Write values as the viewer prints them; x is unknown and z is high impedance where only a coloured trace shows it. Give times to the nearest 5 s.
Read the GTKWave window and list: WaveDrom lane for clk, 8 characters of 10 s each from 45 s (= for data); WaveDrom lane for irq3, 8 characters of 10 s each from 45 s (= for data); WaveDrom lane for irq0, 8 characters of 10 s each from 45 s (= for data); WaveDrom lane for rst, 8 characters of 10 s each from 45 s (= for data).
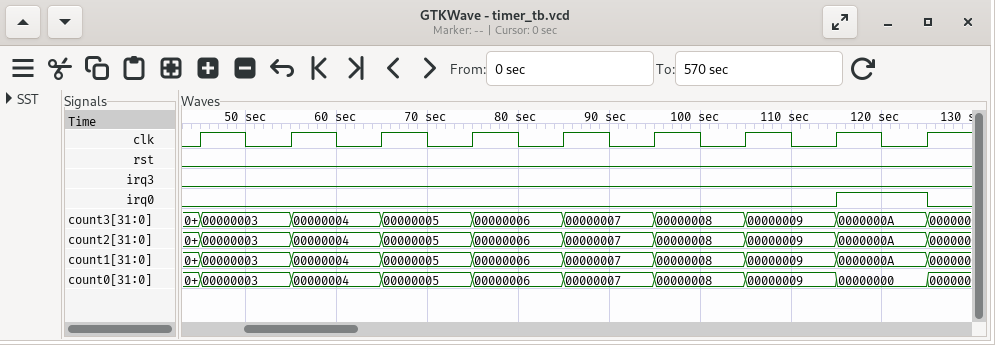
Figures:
{name: 'clk', wave: 'p.......'}
{name: 'irq3', wave: '0.......'}
{name: 'irq0', wave: '0......1'}
{name: 'rst', wave: '0.......'}
